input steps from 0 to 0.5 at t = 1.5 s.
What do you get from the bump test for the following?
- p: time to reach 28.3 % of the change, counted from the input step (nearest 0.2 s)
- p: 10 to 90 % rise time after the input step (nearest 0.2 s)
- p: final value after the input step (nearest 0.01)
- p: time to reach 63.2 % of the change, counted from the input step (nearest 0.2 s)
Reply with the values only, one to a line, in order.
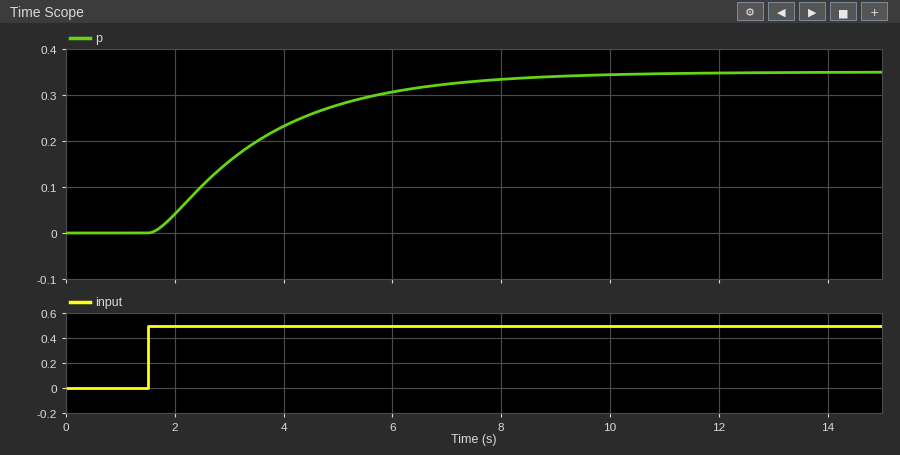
1.0 s
4.4 s
0.35
2.4 s
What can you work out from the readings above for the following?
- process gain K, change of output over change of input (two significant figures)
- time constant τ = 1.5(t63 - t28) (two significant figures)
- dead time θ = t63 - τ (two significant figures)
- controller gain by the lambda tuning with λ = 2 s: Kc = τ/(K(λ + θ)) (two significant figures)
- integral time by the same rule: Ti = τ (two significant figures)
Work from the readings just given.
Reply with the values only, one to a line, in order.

0.70
2.1 s
0.30 s
1.3
2.1 s
